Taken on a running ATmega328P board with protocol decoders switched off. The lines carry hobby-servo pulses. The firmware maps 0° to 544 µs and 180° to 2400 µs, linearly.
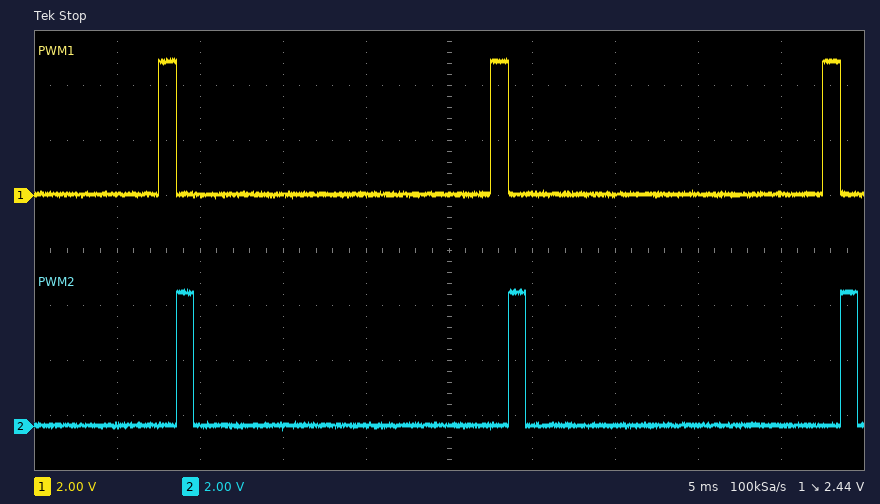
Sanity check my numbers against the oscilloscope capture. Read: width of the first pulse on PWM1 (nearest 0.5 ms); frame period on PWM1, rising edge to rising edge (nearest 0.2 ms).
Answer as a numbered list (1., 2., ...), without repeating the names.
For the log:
1. 1.0 ms
2. 20.0 ms
